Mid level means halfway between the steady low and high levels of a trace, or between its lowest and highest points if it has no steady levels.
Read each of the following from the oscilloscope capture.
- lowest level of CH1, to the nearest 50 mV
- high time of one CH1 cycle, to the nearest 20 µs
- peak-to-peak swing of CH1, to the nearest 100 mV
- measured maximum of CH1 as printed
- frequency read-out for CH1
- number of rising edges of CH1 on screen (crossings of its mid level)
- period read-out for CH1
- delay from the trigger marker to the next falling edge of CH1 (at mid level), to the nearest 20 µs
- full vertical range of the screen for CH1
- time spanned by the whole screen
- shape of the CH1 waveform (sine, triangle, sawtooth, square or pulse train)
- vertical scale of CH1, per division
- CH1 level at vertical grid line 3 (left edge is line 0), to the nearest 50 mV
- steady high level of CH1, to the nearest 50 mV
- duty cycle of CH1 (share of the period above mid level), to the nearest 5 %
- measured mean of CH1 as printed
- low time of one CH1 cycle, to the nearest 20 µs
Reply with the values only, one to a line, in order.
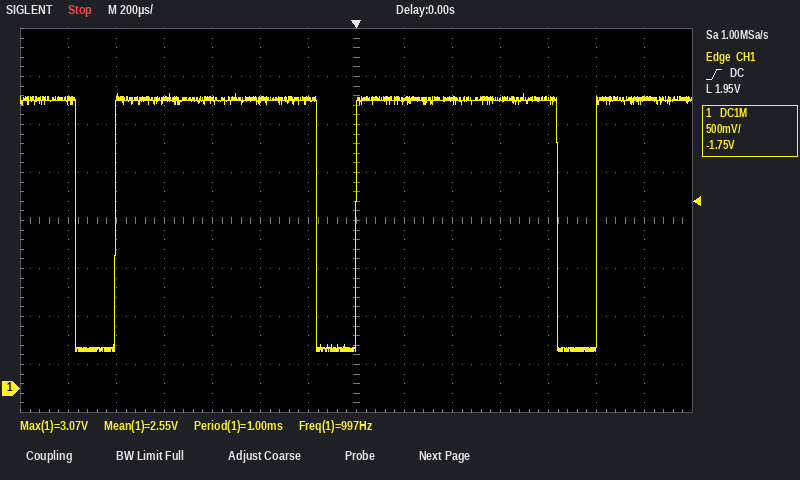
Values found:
400 mV
840 µs
2.70 V
3.07 V
997 Hz
3
1.00 ms
840 µs
4 V
2.8 ms
pulse train
500 mV
3.00 V
3.00 V
85 %
2.55 V
160 µs
